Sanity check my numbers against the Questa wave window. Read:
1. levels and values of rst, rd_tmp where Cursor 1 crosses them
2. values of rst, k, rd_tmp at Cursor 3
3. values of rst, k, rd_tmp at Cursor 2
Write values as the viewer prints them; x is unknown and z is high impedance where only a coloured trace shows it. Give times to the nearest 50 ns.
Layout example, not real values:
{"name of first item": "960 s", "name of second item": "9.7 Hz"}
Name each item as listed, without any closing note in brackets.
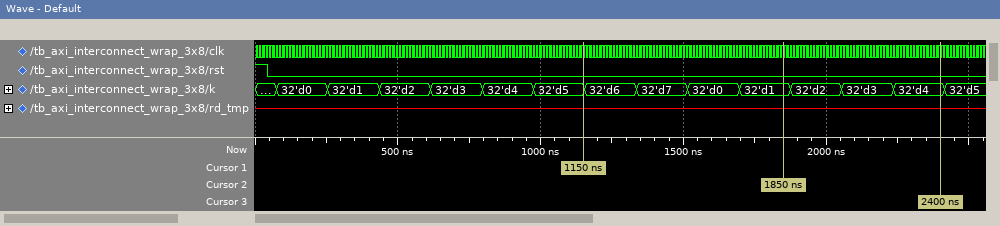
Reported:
{"levels and values of rst, rd_tmp where Cursor 1 crosses them": "rst=0, rd_tmp=x", "values of rst, k, rd_tmp at Cursor 3": "rst=0, k=32'd4, rd_tmp=x", "values of rst, k, rd_tmp at Cursor 2": "rst=0, k=32'd1, rd_tmp=x"}
